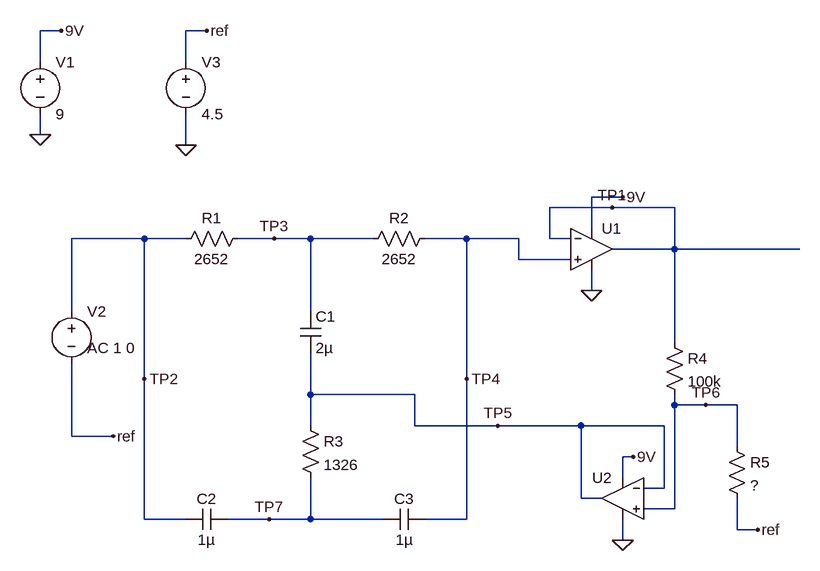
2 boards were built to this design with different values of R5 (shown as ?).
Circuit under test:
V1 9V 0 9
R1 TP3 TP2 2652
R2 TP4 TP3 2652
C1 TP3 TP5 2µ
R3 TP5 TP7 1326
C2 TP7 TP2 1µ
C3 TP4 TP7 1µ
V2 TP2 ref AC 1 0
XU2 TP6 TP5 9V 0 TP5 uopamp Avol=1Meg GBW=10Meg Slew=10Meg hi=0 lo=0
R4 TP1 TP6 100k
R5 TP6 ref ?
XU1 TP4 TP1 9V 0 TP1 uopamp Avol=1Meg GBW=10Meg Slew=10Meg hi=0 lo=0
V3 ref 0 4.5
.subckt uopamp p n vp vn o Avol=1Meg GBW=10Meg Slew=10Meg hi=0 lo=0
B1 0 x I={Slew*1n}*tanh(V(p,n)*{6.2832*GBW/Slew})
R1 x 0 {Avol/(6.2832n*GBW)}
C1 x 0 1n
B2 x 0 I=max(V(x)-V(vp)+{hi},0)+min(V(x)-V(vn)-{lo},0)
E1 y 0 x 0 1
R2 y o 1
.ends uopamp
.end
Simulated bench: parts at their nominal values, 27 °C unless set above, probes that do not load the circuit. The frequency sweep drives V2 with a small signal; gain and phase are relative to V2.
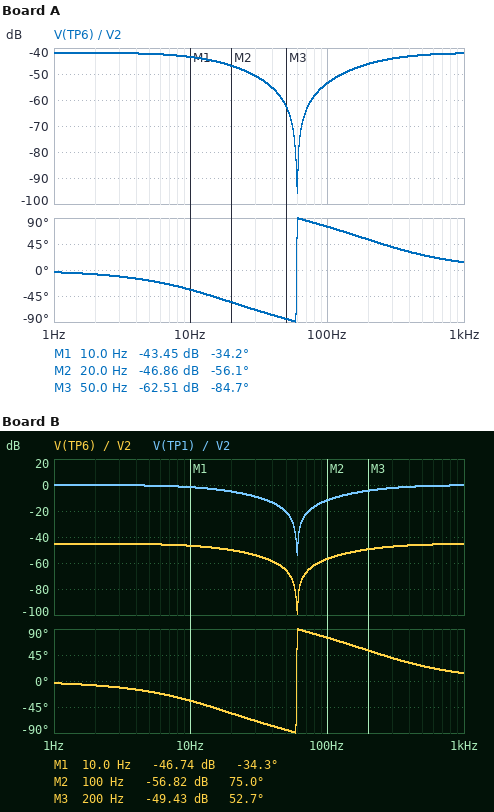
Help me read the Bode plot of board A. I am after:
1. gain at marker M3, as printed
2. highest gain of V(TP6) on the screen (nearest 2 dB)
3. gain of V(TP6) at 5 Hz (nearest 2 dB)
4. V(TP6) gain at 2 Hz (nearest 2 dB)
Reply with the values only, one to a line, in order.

-62.51 dB
-42 dB
-42 dB
-42 dB
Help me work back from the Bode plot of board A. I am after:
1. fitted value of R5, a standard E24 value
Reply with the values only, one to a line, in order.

820 Ω
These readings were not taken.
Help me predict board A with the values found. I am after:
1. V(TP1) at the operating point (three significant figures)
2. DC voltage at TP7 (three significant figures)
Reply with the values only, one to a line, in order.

4.50 V
4.50 V
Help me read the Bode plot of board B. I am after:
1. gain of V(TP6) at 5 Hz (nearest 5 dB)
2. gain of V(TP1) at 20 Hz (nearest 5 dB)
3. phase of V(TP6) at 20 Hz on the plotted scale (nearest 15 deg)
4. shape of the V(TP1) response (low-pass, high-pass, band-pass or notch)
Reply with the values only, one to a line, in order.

-45 dB
-5 dB
-60 deg
notch
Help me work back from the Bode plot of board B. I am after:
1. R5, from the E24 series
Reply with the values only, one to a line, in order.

560 Ω
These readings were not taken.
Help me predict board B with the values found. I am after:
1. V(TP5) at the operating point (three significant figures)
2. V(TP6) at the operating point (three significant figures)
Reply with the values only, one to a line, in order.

4.50 V
4.50 V
